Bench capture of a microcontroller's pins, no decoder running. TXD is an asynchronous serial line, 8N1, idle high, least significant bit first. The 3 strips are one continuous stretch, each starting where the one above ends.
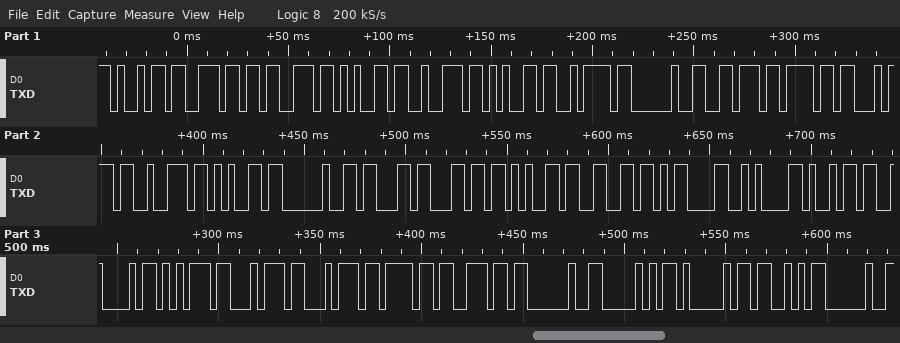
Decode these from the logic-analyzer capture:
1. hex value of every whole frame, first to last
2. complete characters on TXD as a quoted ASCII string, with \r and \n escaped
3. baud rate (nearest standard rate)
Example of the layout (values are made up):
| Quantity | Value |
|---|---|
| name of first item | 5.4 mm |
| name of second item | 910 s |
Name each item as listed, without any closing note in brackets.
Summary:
| Quantity | Value |
|---|---|
| hex value of every whole frame, first to last | 69 6E 73 65 72 65 7A 20 76 6F 74 72 65 20 63 6C 65 66 0D 0A 69 42 75 74 74 6F 6E 20 50 41 53 20 |
| complete characters on TXD as a quoted ASCII string, with \r and \n escaped | "inserez votre clef\r\niButton PAS " |
| baud rate | 300 baud |
